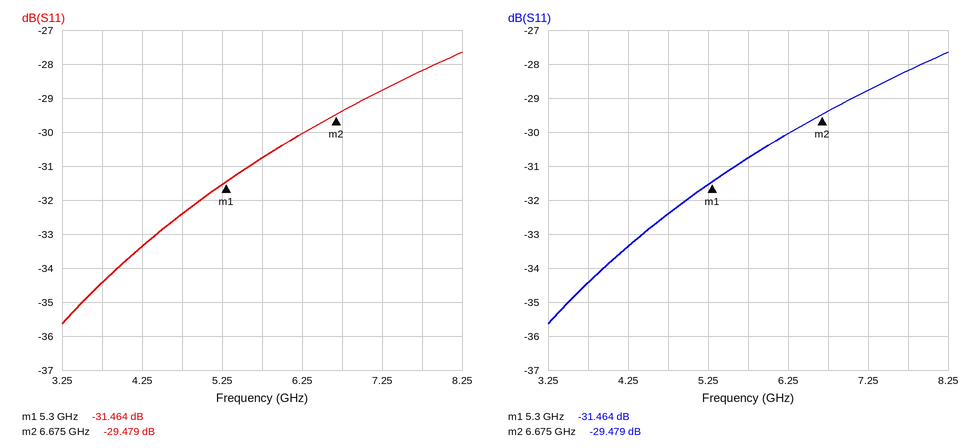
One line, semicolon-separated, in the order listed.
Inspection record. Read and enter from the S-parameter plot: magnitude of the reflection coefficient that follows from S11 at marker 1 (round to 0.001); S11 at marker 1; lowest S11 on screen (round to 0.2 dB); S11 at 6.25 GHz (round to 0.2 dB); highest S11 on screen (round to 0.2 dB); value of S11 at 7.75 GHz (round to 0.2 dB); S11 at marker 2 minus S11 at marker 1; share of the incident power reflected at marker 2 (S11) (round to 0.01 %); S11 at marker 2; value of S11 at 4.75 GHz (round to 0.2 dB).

0.027; -31.464 dB; -35.6 dB; -30.0 dB; -27.6 dB; -28.2 dB; 1.985 dB; 0.11 %; -29.479 dB; -32.4 dB
